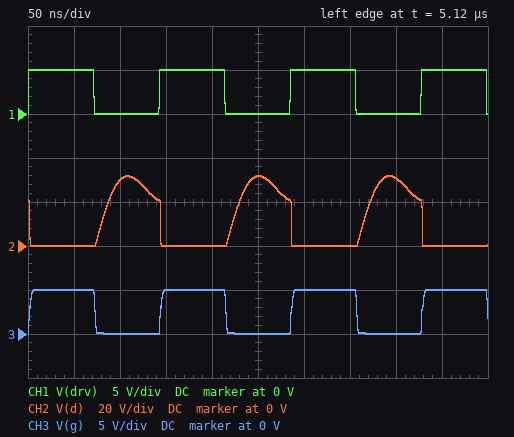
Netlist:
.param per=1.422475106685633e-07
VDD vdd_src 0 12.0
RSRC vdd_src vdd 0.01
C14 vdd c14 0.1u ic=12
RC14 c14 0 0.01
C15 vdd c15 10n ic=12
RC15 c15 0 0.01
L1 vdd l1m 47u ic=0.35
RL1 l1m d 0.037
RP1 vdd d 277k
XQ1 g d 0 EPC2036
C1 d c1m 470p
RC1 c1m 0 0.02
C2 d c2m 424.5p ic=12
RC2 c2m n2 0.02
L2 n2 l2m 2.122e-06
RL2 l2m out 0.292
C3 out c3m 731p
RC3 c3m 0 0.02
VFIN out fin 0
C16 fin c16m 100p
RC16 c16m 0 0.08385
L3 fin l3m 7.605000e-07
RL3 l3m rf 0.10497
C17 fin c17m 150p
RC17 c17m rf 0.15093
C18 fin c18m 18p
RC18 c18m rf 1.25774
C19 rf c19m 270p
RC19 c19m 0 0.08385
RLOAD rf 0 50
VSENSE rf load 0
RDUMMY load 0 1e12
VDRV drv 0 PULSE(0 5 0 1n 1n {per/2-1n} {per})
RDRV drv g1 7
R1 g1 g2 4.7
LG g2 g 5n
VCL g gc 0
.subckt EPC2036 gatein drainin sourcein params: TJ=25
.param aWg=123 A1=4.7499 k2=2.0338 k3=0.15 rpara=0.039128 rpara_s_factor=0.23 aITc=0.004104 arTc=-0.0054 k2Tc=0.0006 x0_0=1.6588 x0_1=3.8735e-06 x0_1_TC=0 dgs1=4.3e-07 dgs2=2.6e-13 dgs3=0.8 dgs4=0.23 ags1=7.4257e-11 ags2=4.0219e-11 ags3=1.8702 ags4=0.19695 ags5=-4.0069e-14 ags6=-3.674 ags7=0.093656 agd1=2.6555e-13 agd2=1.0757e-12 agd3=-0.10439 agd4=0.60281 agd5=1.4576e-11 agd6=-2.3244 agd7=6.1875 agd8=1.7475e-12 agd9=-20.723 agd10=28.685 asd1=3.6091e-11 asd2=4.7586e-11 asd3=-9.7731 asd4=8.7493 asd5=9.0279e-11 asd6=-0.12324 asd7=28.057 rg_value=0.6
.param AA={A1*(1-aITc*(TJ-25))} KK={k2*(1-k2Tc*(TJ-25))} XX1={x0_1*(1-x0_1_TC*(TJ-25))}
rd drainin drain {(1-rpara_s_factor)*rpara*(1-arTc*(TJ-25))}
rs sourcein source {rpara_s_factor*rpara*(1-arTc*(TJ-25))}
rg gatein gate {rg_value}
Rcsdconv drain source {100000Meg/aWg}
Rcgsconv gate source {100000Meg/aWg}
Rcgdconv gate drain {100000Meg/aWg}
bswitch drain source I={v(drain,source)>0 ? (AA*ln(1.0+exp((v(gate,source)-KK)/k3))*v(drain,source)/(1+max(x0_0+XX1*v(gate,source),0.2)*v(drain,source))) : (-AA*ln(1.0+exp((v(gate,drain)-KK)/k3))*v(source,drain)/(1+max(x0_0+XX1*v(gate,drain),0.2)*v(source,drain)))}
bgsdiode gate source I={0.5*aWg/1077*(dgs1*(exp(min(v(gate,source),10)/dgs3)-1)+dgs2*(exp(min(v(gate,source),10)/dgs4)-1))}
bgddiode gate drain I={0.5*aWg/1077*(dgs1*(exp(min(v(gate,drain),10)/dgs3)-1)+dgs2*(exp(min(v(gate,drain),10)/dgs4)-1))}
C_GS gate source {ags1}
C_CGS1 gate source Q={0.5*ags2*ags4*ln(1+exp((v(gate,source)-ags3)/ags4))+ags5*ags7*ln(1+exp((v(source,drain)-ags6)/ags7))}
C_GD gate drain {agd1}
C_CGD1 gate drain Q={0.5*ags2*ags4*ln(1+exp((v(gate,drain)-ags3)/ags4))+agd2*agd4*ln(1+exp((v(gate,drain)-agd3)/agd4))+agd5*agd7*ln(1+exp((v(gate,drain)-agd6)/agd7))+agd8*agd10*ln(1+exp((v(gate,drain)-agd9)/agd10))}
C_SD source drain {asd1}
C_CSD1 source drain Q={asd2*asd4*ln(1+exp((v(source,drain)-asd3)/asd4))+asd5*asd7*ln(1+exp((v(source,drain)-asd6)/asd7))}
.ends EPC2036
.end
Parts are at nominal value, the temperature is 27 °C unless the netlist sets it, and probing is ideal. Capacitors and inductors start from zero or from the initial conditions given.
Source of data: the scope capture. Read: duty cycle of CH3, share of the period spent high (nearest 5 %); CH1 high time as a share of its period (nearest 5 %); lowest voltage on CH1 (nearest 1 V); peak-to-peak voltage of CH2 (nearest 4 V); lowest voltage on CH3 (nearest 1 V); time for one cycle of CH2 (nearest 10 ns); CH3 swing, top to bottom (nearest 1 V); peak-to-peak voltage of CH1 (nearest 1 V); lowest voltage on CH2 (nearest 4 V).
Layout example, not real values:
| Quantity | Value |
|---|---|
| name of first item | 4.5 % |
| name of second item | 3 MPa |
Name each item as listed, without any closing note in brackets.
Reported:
| Quantity | Value |
|---|---|
| duty cycle of CH3, share of the period spent high | 50 % |
| CH1 high time as a share of its period | 50 % |
| lowest voltage on CH1 | 0 V |
| peak-to-peak voltage of CH2 | 32 V |
| lowest voltage on CH3 | 0 V |
| time for one cycle of CH2 | 140 ns |
| CH3 swing, top to bottom | 5 V |
| peak-to-peak voltage of CH1 | 5 V |
| lowest voltage on CH2 | 0 V |
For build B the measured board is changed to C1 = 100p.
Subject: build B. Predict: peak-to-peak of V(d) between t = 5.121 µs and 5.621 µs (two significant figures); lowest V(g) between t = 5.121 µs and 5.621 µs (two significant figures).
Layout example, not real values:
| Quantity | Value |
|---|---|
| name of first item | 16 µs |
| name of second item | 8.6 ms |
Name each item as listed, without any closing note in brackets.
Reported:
| Quantity | Value |
|---|---|
| peak-to-peak of V(d) between t = 5.121 µs and 5.621 µs | 50 V |
| lowest V(g) between t = 5.121 µs and 5.621 µs | -80 mV |
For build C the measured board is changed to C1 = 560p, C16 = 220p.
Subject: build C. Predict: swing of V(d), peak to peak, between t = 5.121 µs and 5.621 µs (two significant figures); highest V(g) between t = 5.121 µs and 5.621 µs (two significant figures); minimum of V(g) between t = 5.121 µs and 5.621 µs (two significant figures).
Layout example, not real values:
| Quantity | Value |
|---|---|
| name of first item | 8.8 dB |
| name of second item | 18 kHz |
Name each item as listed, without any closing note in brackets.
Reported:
| Quantity | Value |
|---|---|
| swing of V(d), peak to peak, between t = 5.121 µs and 5.621 µs | 33 V |
| highest V(g) between t = 5.121 µs and 5.621 µs | 5.0 V |
| minimum of V(g) between t = 5.121 µs and 5.621 µs | -10 mV |
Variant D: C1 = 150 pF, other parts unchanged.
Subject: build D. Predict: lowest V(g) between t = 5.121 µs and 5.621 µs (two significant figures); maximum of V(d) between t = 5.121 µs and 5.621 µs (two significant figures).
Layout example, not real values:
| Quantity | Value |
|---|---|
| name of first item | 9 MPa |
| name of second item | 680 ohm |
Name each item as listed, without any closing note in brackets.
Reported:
| Quantity | Value |
|---|---|
| lowest V(g) between t = 5.121 µs and 5.621 µs | -48 mV |
| maximum of V(d) between t = 5.121 µs and 5.621 µs | 44 V |
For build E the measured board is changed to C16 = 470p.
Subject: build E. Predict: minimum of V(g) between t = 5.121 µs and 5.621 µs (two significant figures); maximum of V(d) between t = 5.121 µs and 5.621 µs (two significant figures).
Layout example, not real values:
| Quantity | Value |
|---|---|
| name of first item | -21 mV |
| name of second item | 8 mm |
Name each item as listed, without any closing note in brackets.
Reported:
| Quantity | Value |
|---|---|
| minimum of V(g) between t = 5.121 µs and 5.621 µs | -48 mV |
| maximum of V(d) between t = 5.121 µs and 5.621 µs | 36 V |
